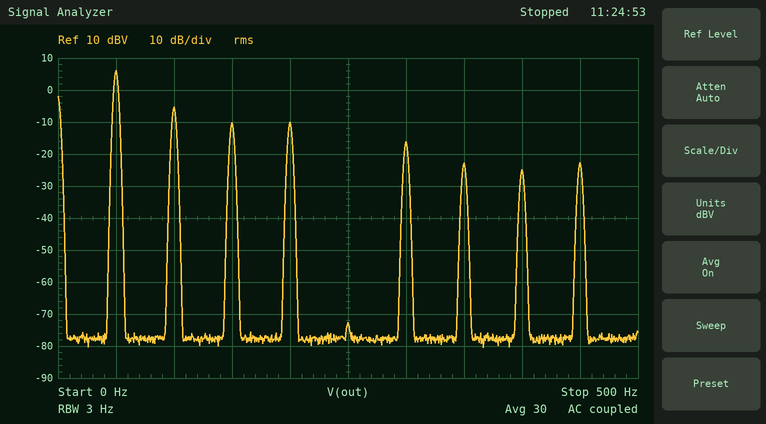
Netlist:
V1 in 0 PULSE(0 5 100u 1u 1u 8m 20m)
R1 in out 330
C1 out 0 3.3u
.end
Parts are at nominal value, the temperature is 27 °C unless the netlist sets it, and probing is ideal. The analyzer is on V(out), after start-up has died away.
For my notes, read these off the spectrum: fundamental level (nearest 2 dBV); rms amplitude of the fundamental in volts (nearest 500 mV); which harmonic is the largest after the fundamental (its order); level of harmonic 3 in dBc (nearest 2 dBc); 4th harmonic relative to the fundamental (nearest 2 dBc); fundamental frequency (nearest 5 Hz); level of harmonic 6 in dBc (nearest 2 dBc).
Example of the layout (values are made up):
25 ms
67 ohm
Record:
6 dBV
2.0 V
2
-16 dBc
-16 dBc
50 Hz
-22 dBc
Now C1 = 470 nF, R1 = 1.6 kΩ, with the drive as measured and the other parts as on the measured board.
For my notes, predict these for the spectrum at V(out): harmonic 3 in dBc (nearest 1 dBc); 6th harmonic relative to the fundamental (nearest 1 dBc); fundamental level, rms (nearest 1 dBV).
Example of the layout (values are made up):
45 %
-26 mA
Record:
-15 dBc
-20 dBc
6 dBV
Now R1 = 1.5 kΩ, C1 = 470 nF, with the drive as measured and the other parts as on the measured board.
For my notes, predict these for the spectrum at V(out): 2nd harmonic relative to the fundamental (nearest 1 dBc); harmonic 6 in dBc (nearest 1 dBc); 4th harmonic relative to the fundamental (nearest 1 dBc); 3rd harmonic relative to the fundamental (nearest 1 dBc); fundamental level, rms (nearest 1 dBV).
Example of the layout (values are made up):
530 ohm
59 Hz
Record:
-11 dBc
-20 dBc
-14 dBc
-15 dBc
6 dBV
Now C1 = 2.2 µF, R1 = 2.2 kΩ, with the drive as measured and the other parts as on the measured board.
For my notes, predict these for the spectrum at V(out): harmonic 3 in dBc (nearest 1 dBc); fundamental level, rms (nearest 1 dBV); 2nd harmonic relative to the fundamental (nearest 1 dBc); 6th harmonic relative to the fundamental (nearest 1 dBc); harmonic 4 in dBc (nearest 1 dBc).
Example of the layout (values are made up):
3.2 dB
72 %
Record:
-22 dBc
1 dBV
-15 dBc
-30 dBc
-23 dBc
